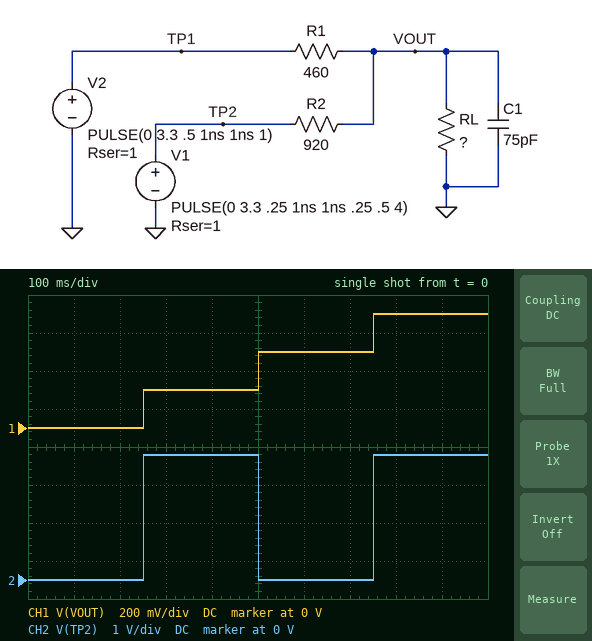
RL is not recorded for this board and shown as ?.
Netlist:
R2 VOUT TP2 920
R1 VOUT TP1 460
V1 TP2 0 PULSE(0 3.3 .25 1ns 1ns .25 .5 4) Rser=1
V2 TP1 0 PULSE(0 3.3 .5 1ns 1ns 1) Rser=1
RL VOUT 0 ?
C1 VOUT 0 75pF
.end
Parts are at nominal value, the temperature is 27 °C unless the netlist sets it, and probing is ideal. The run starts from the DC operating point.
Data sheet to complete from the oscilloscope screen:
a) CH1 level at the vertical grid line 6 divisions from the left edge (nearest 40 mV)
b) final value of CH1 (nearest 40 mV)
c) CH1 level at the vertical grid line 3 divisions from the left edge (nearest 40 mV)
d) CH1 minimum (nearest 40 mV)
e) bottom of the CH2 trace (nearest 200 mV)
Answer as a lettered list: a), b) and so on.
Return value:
a) 400 mV
b) 600 mV
c) 200 mV
d) 0 V
e) 0 V
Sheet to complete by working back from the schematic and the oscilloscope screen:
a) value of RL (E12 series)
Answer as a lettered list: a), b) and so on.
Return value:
a) 68 Ω
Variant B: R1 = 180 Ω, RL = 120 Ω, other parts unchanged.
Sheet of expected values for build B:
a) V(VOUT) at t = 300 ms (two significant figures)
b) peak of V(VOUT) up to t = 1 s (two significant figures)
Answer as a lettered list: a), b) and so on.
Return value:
a) 240 mV
b) 1.5 V
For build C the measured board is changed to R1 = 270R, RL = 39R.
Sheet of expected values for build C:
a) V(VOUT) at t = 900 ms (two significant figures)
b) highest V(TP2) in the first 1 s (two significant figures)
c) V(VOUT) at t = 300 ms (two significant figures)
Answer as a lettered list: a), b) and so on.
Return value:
a) 520 mV
b) 3.3 V
c) 120 mV
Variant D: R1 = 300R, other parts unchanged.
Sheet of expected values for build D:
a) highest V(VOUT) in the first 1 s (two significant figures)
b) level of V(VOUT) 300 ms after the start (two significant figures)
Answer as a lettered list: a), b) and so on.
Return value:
a) 760 mV
b) 190 mV
